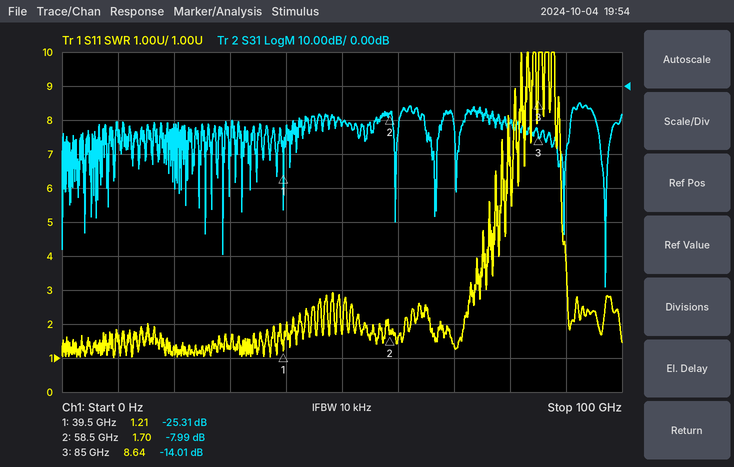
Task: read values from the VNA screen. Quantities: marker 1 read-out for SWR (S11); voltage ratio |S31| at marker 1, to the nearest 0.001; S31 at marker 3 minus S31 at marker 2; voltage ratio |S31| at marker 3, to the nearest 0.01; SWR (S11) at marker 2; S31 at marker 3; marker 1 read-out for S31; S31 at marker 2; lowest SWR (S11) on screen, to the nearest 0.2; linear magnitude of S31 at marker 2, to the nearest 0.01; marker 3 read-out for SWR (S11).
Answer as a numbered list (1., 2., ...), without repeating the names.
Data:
1. 1.21
2. 0.054
3. -6.02 dB
4. 0.20
5. 1.70
6. -14.01 dB
7. -25.31 dB
8. -7.99 dB
9. 1.0
10. 0.40
11. 8.64
